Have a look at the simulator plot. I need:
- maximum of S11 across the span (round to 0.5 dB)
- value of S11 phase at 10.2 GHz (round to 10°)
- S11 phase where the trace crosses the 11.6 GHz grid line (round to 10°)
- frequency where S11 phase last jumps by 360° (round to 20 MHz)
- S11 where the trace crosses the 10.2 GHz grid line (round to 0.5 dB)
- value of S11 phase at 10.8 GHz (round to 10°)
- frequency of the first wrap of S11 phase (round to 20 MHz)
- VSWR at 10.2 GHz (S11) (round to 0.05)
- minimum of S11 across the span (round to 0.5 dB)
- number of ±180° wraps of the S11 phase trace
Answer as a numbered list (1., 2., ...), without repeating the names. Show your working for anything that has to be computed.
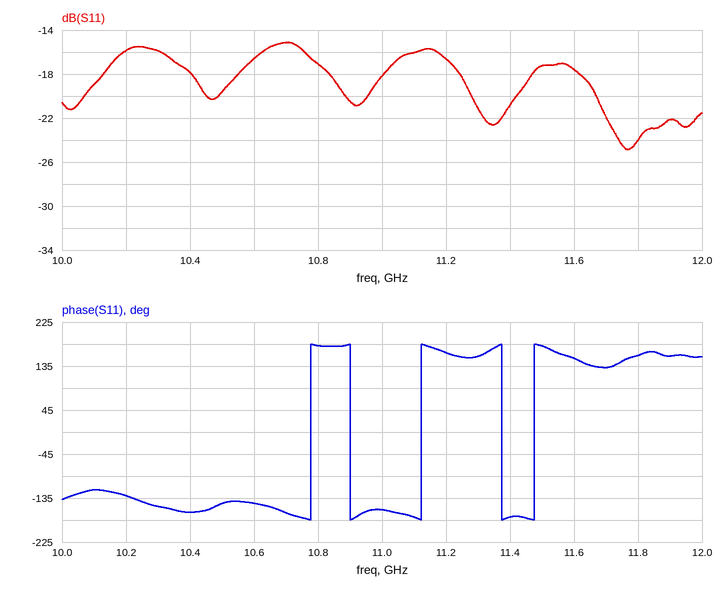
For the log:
1. -15.0 dB
2. -130°
3. 150°
4. 11.48 GHz
5. -16.0 dB
6. 180°
7. 10.78 GHz
8. |Γ| = 10^(-16/20) = 0.1585; VSWR = (1 + 0.1585)/(1 − 0.1585) ≈ 1.38, so 1.40 to the nearest 0.05
9. -25.0 dB
10. 5
